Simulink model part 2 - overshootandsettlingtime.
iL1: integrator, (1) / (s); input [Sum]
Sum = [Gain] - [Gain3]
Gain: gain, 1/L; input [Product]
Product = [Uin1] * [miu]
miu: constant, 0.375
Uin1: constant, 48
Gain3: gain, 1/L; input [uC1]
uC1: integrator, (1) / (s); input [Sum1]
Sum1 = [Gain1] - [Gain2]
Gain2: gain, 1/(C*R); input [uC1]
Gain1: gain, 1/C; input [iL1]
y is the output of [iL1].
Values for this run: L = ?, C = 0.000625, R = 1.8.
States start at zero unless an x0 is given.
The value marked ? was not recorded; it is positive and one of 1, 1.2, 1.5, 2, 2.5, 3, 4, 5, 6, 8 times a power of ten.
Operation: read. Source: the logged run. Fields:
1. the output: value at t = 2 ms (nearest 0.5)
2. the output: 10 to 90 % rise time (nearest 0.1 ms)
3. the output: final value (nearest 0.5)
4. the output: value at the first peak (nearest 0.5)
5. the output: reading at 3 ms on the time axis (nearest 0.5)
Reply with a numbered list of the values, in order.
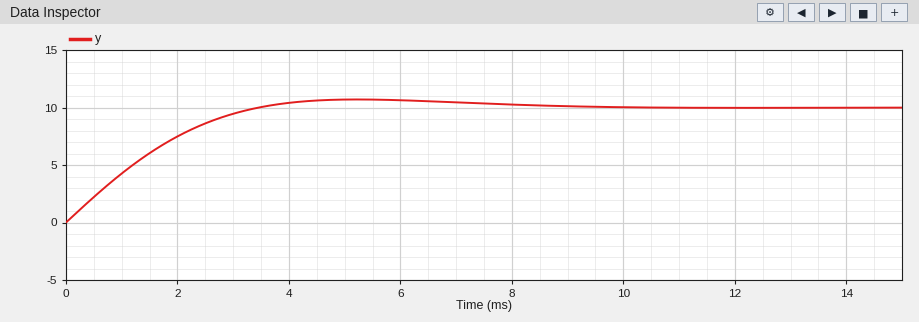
1. 7.5
2. 2.5 ms
3. 10.0
4. 10.5
5. 9.5
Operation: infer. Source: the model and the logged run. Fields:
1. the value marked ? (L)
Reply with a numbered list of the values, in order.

1. 0.004
